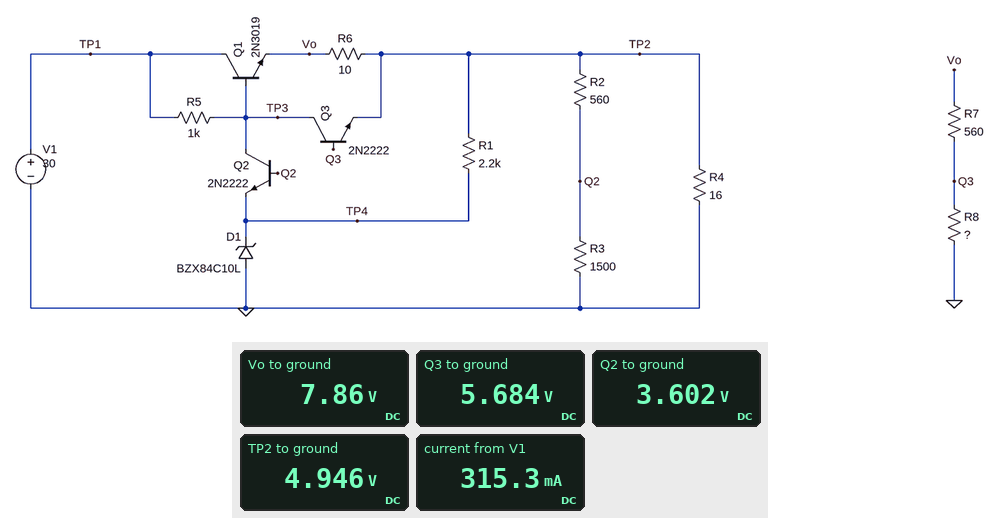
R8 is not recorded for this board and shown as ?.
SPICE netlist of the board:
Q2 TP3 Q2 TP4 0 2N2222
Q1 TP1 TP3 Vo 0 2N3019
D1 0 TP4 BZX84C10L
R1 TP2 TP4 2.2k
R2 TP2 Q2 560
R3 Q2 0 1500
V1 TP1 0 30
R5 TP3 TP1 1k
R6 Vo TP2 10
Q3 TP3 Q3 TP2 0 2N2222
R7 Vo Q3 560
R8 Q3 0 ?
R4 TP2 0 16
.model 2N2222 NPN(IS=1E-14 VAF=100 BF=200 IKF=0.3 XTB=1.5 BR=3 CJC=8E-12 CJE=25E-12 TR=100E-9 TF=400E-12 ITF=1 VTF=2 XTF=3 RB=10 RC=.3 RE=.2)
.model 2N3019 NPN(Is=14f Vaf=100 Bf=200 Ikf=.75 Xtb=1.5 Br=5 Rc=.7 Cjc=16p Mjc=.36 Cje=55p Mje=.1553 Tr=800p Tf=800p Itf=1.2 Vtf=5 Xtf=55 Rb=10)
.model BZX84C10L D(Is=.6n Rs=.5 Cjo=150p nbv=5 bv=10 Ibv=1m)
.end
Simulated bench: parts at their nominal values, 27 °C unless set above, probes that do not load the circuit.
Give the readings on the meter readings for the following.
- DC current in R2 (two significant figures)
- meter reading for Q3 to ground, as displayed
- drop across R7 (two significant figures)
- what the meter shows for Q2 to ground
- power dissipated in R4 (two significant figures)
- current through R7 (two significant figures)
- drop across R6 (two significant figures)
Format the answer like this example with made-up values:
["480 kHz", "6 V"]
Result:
["2.4 mA", "5.684 V", "2.2 V", "3.602 V", "1.5 W", "3.9 mA", "2.9 V"]
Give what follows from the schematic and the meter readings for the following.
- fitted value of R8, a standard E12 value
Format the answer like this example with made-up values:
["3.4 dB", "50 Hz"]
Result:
["1.5 kΩ"]
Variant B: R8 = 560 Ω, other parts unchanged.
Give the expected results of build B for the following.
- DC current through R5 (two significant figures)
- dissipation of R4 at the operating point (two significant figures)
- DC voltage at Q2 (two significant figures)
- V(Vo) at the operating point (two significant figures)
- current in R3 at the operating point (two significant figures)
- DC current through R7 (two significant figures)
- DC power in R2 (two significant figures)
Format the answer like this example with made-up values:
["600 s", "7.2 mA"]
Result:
["7.9 mA", "11 W", "9.5 V", "21 V", "6.3 mA", "19 mA", "22 mW"]
